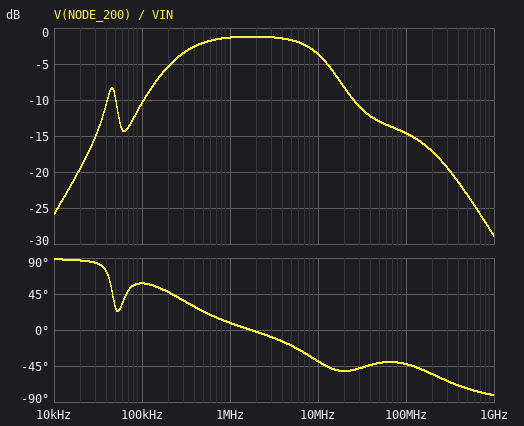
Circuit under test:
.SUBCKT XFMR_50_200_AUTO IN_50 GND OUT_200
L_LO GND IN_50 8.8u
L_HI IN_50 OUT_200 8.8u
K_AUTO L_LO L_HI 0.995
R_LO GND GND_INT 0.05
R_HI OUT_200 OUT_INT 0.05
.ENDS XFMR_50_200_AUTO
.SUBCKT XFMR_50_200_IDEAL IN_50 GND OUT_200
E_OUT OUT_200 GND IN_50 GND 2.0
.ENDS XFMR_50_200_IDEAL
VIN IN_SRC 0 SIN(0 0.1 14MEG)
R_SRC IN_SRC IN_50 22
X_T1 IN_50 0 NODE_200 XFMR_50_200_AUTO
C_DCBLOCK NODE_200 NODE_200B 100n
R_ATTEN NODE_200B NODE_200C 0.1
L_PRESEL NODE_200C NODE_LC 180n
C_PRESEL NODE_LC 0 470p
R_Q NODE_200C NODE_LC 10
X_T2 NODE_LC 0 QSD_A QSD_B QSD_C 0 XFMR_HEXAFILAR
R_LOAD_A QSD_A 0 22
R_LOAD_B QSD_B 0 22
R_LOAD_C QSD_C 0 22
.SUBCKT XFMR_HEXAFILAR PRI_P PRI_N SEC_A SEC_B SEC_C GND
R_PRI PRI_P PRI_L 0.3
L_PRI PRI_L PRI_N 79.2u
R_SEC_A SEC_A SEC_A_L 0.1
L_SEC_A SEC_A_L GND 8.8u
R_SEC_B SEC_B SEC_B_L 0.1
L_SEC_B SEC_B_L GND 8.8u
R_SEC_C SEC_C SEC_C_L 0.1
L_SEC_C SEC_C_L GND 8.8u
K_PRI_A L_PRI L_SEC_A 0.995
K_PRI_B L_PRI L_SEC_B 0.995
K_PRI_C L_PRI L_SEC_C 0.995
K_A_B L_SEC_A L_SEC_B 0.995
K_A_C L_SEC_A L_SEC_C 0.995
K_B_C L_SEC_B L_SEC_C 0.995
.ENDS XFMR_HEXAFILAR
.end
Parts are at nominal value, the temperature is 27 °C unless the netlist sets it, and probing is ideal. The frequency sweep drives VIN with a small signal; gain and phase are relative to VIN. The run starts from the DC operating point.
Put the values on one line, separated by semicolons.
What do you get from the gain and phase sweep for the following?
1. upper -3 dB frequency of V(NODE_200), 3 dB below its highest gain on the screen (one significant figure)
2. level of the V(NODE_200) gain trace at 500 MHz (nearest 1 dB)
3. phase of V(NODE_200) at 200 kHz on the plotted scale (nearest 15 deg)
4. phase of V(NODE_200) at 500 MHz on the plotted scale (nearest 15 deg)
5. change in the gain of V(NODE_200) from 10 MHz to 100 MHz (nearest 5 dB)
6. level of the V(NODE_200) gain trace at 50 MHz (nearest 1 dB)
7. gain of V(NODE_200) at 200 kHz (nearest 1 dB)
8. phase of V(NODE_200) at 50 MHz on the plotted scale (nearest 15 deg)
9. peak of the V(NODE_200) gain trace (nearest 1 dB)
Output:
10 MHz; -23 dB; 45 deg; -75 deg; -10 dB; -13 dB; -5 dB; -45 deg; -1 dB
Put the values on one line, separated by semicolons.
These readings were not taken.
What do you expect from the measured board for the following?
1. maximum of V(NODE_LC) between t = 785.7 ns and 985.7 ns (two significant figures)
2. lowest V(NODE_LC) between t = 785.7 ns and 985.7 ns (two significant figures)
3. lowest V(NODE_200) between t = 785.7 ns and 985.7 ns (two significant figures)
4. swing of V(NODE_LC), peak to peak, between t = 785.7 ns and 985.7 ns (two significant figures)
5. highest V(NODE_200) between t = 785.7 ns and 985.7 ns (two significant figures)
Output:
54 mV; -55 mV; -53 mV; 110 mV; 52 mV
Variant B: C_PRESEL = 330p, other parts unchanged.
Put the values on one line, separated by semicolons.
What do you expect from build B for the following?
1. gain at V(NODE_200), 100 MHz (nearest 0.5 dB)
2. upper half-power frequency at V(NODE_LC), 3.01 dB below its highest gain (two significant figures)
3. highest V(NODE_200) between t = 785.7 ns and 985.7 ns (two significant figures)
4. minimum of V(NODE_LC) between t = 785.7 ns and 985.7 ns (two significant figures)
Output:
-14.0 dB; 18 MHz; 72 mV; -73 mV
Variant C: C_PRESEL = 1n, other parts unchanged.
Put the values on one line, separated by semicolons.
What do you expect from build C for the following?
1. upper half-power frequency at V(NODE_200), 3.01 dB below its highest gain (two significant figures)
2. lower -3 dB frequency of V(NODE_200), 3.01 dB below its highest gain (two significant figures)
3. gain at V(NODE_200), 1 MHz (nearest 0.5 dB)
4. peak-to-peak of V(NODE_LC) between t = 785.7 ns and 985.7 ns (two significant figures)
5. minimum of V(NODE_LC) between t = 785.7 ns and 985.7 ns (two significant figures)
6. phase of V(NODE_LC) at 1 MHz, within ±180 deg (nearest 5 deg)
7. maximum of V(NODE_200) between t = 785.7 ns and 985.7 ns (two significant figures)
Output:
4.5 MHz; 240 kHz; -1.0 dB; 51 mV; -26 mV; 0 deg; 24 mV
